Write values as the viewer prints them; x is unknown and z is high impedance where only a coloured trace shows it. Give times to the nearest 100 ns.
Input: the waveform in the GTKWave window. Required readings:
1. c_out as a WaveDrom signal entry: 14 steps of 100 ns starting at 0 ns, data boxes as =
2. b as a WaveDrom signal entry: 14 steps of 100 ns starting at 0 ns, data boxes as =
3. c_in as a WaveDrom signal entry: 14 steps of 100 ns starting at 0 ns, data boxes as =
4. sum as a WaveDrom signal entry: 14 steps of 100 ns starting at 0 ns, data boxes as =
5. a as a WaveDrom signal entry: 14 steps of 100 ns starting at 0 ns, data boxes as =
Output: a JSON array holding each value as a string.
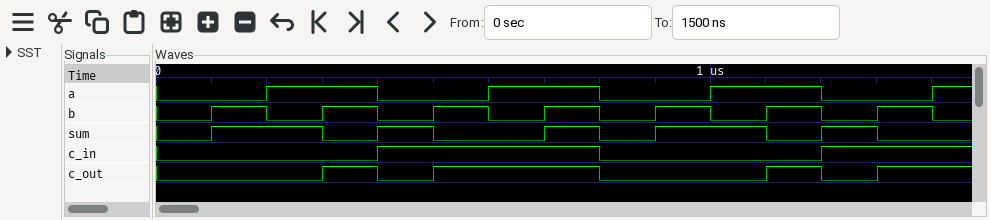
["{name: 'c_out', wave: '0..101..0..101'}", "{name: 'b', wave: '01010101010101'}", "{name: 'c_in', wave: '0...1...0...1.'}", "{name: 'sum', wave: '01.010.101.010'}", "{name: 'a', wave: '0.1.0.1.0.1.0.'}"]
